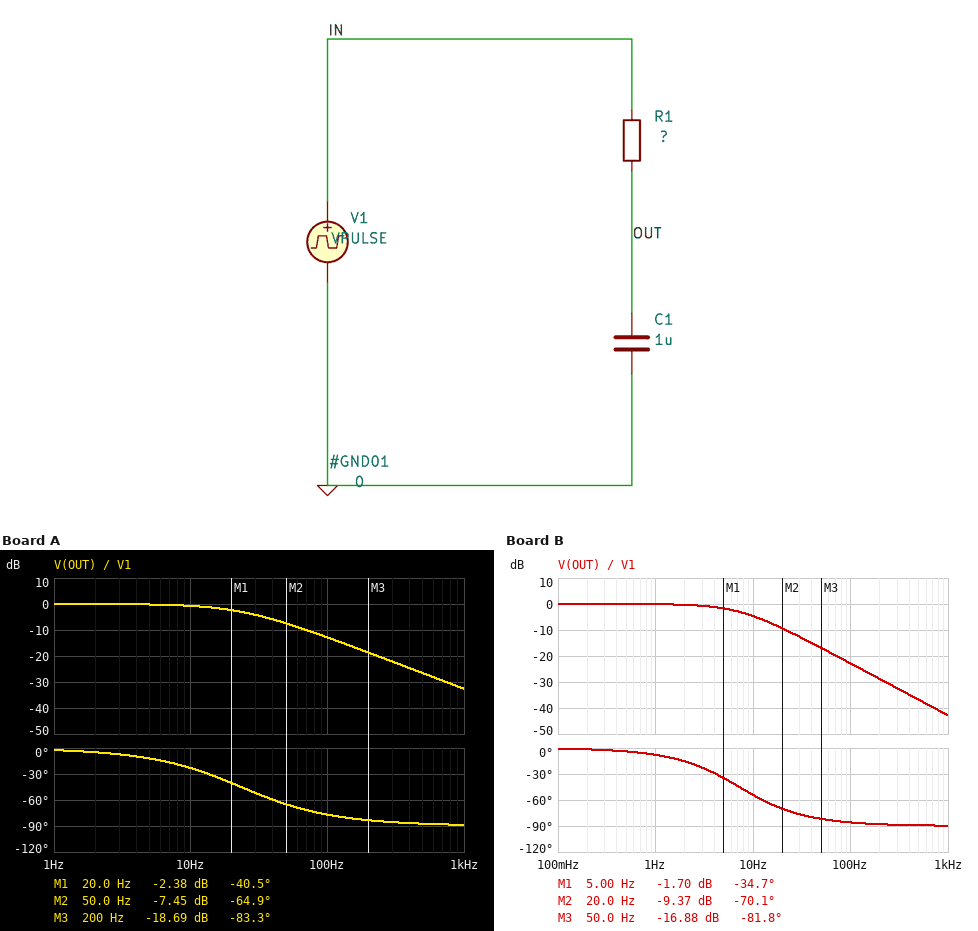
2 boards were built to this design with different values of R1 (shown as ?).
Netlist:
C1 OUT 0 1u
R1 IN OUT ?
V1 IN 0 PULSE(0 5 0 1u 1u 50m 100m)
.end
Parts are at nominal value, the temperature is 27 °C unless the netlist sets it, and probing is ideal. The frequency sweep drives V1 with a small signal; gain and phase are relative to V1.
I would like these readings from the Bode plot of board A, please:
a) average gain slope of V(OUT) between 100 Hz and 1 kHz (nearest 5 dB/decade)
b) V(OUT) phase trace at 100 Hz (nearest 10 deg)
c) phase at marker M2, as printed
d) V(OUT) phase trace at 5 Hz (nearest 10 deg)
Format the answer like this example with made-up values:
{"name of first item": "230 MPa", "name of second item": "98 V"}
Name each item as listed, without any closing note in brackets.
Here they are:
{"average gain slope of V(OUT) between 100 Hz and 1 kHz": "-20 dB/decade", "V(OUT) phase trace at 100 Hz": "-80 deg", "phase at marker M2, as printed": "-64.9 deg", "V(OUT) phase trace at 5 Hz": "-10 deg"}
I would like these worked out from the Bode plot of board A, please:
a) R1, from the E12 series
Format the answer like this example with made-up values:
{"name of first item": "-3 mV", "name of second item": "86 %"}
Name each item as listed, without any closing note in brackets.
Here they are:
{"R1, from the E12 series": "6.8 kΩ"}
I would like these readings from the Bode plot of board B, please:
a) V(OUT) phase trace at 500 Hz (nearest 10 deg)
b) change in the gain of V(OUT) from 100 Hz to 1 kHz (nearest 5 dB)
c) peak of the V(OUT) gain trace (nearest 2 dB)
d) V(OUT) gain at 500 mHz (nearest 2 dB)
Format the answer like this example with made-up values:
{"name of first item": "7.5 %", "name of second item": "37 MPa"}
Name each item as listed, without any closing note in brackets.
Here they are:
{"V(OUT) phase trace at 500 Hz": "-90 deg", "change in the gain of V(OUT) from 100 Hz to 1 kHz": "-20 dB", "peak of the V(OUT) gain trace": "0 dB", "V(OUT) gain at 500 mHz": "0 dB"}
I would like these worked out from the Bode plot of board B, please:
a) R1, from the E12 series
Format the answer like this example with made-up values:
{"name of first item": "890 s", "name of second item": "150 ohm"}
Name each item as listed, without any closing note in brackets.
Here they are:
{"R1, from the E12 series": "22 kΩ"}
